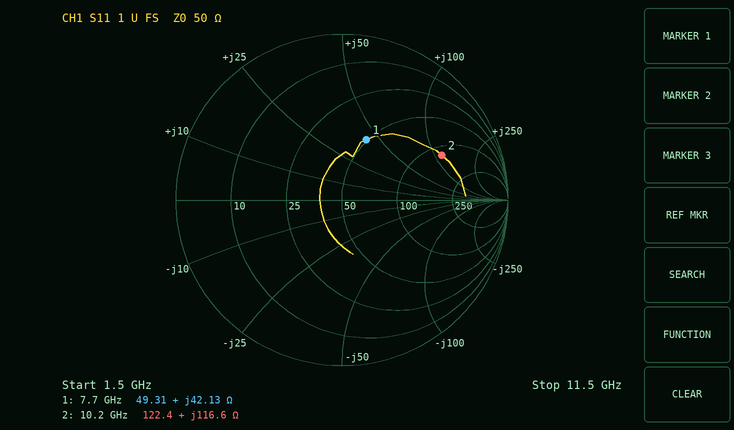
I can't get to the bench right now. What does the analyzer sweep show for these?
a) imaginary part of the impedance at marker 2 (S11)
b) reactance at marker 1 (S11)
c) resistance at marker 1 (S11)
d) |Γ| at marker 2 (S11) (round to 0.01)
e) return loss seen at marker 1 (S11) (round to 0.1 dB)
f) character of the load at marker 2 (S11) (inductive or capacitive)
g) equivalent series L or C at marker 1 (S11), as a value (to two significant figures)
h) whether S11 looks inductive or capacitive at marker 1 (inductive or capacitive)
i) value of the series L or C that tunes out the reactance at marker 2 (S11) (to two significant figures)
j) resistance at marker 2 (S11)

+116.6 Ω
+42.13 Ω
49.31 Ω
0.66
8.2 dB
inductive
870 pH
inductive
130 fF
122.4 Ω
